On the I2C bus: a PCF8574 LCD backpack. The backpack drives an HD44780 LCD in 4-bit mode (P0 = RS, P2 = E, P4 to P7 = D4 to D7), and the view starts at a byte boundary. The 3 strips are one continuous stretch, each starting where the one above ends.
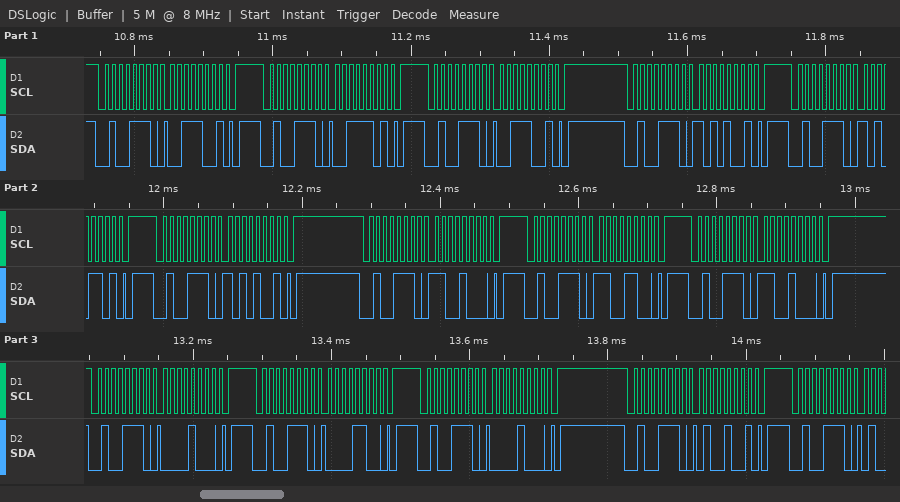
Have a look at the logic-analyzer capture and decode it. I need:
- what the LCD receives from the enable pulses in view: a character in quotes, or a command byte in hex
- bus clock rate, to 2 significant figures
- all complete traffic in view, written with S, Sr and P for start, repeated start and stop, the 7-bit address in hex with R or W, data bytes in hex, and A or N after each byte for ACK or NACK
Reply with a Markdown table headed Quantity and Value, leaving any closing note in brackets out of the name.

| Quantity | Value |
|---|---|
| what the LCD receives from the enable pulses in view: a character in quotes, or a command byte in hex | ':' 0xC0 |
| bus clock rate, to 2 significant figures | 100 kHz |
| all complete traffic in view, written with S, Sr and P for start, repeated start and stop, the 7-bit address in hex with R or W, data bytes in hex, and A or N after each byte for ACK or NACK | S 27W A 39 A P S 27W A 3D A P S 27W A 39 A P S 27W A A9 A P S 27W A AD A P S 27W A A9 A P S 27W A C8 A P S 27W A CC A P S 27W A C8 A P S 27W A 08 A P S 27W A 0C A P S 27W A 08 A P S 27W A 49 A P S 27W A |
